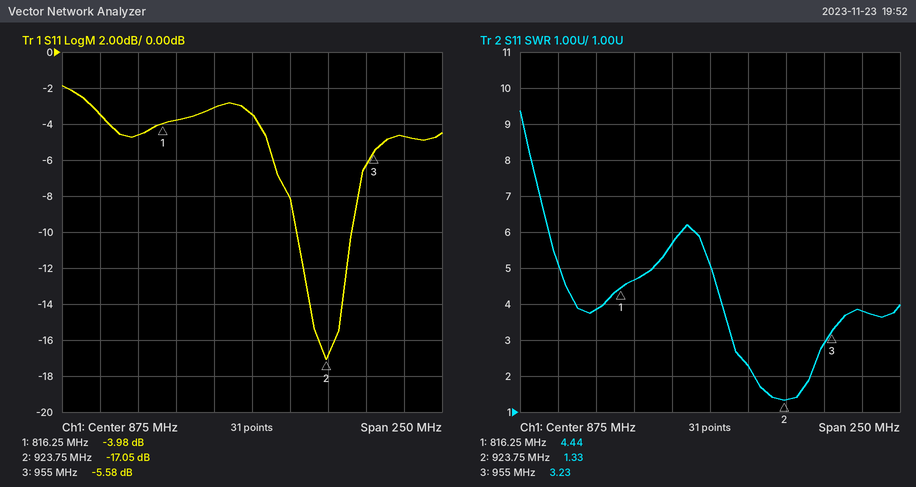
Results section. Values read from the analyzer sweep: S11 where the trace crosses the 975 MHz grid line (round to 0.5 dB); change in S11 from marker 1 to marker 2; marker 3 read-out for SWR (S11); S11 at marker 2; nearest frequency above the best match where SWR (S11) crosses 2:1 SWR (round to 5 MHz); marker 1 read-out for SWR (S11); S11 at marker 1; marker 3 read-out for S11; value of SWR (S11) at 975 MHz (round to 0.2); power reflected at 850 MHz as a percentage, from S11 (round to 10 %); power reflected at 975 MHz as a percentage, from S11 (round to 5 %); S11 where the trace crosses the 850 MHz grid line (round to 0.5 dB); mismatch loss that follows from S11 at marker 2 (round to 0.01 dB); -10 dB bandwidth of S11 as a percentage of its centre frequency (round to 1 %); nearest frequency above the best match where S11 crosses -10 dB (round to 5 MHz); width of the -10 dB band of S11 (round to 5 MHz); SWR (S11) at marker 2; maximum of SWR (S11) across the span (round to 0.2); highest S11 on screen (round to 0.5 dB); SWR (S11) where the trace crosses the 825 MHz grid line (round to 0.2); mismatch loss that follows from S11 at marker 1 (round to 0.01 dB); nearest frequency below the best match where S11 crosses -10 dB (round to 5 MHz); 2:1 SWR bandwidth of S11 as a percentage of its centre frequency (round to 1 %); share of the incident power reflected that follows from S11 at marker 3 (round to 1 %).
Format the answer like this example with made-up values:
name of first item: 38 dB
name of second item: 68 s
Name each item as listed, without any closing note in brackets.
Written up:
S11 where the trace crosses the 975 MHz grid line: -4.5 dB
change in S11 from marker 1 to marker 2: -13.07 dB
marker 3 read-out for SWR: 3.23
S11 at marker 2: -17.05 dB
nearest frequency above the best match where SWR (S11) crosses 2:1 SWR: 940 MHz
marker 1 read-out for SWR: 4.44
S11 at marker 1: -3.98 dB
marker 3 read-out for S11: -5.58 dB
value of SWR (S11) at 975 MHz: 3.8
power reflected at 850 MHz as a percentage, from S11: 50 %
power reflected at 975 MHz as a percentage, from S11: 35 %
S11 where the trace crosses the 850 MHz grid line: -3.0 dB
mismatch loss that follows from S11 at marker 2: 0.09 dB
-10 dB bandwidth of S11 as a percentage of its centre frequency: 4 %
nearest frequency above the best match where S11 crosses -10 dB: 940 MHz
width of the -10 dB band of S11: 35 MHz
SWR (S11) at marker 2: 1.33
maximum of SWR (S11) across the span: 9.4
highest S11 on screen: -2.0 dB
SWR (S11) where the trace crosses the 825 MHz grid line: 4.6
mismatch loss that follows from S11 at marker 1: 2.22 dB
nearest frequency below the best match where S11 crosses -10 dB: 905 MHz
2:1 SWR bandwidth of S11 as a percentage of its centre frequency: 4 %
share of the incident power reflected that follows from S11 at marker 3: 28 %
